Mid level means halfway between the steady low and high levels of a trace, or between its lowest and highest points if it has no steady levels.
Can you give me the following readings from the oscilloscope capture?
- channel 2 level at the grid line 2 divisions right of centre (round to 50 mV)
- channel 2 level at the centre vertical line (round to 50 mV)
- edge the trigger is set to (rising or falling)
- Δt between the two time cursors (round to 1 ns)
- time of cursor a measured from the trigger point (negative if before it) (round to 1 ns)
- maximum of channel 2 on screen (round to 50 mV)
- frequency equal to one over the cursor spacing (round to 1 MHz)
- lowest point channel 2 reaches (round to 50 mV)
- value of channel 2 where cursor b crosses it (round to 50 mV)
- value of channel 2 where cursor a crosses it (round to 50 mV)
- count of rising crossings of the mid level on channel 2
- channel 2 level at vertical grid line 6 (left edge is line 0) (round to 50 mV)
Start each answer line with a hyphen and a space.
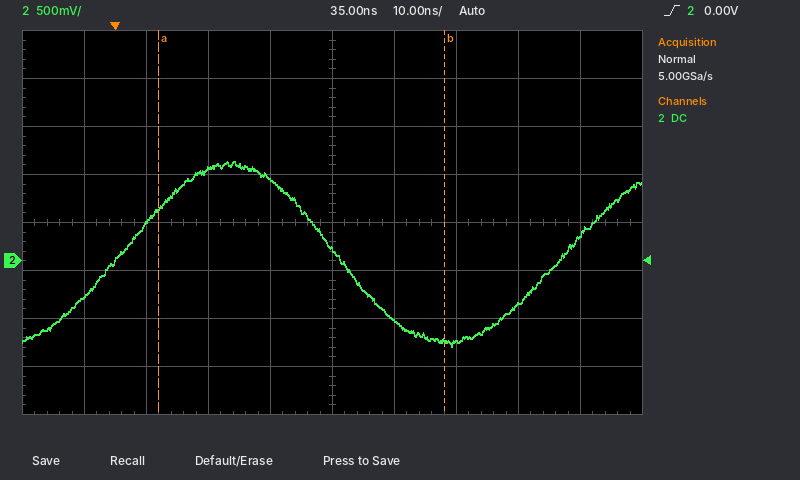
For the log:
- -850 mV
- 100 mV
- rising
- 46 ns
- +7 ns
- 1.05 V
- 22 MHz
- -900 mV
- -850 mV
- 550 mV
- 2
- -600 mV
